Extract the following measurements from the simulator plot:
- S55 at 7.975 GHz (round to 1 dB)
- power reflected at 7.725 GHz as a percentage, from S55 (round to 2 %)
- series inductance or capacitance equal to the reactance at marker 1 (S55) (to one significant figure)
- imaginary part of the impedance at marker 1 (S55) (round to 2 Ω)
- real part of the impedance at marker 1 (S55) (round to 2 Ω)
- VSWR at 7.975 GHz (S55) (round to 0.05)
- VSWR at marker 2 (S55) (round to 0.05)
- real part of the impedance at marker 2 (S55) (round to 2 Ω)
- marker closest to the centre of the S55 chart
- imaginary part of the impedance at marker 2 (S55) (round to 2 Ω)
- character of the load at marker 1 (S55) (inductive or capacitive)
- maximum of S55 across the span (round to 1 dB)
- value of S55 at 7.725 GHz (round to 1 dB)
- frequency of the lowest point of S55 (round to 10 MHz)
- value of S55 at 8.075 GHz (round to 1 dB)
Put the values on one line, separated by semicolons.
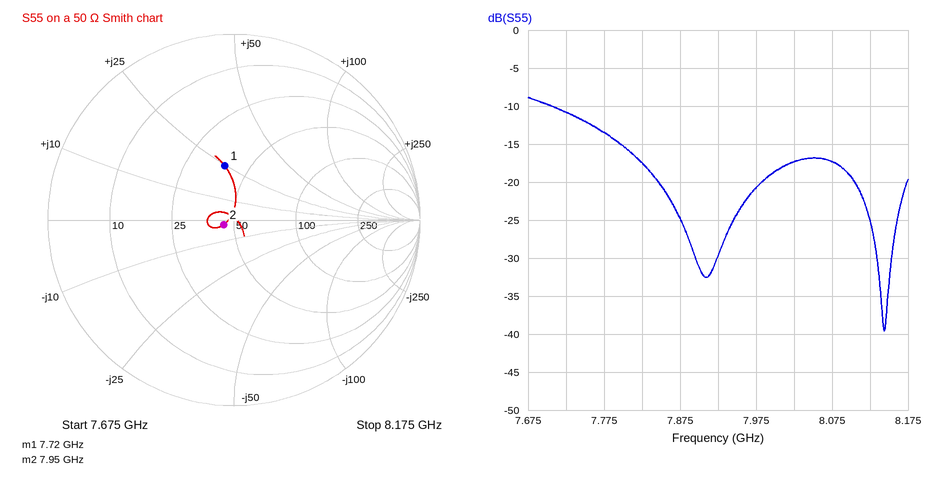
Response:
-21 dB; 8 %; 500 pH; +24 Ω; 38 Ω; 1.20; 1.15; 44 Ω; marker 2; -2 Ω; inductive; -9 dB; -11 dB; 8.14 GHz; -17 dB
